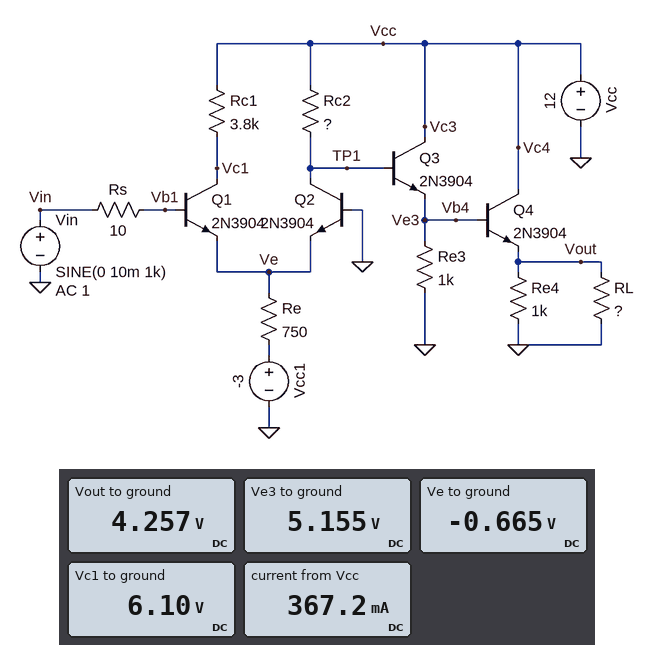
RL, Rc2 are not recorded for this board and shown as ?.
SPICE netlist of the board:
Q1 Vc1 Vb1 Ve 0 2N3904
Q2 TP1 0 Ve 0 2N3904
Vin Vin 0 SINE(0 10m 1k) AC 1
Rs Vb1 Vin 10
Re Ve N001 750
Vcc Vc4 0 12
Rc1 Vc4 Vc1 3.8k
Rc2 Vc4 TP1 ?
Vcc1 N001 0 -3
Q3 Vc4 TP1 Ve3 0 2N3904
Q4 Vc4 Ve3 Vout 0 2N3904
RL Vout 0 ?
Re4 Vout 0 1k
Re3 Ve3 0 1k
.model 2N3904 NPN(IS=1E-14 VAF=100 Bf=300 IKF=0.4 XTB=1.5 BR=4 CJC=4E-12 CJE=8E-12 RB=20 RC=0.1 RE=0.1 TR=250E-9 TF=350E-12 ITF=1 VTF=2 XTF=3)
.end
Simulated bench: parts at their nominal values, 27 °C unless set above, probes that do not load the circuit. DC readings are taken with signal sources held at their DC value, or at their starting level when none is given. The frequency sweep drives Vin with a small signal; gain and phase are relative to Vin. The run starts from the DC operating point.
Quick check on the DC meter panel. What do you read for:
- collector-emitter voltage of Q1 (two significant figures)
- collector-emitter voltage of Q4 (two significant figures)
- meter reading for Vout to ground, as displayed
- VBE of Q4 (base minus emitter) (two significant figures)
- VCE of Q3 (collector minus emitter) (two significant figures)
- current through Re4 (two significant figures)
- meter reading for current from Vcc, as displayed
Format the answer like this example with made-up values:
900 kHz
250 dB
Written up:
6.8 V
7.7 V
4.257 V
900 mV
6.8 V
4.3 mA
367.2 mA
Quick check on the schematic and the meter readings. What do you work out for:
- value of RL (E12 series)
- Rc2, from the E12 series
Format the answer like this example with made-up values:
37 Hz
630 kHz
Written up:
12 Ω
3.9 kΩ
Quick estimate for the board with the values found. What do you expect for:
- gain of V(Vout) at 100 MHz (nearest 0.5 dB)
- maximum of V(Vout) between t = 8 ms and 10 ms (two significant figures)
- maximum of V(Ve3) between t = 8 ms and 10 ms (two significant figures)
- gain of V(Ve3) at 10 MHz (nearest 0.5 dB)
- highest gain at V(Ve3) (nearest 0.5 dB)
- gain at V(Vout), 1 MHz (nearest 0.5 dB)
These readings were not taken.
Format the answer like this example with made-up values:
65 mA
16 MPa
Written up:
4.5 dB
5.3 V
6.2 V
35.0 dB
40.5 dB
40.0 dB
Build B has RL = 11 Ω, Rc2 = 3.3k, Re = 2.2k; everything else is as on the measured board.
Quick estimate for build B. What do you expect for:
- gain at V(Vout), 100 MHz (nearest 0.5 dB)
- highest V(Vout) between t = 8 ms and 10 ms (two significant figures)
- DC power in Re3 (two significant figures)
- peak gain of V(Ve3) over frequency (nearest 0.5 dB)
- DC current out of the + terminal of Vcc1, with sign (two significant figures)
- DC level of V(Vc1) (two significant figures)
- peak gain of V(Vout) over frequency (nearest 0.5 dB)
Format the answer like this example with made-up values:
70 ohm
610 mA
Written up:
-9.5 dB
8.6 V
87 mW
30.0 dB
-1.1 mA
10 V
29.5 dB
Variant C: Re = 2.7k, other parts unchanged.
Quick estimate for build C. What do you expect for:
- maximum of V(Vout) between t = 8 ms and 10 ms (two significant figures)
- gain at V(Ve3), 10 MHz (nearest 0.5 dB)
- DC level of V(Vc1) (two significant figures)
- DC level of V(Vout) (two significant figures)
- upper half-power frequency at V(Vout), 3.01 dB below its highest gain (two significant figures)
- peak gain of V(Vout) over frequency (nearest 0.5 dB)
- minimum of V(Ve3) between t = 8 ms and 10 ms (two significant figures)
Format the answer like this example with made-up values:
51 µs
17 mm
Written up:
8.6 V
25.5 dB
10 V
8.3 V
8.4 MHz
29.5 dB
9.1 V
